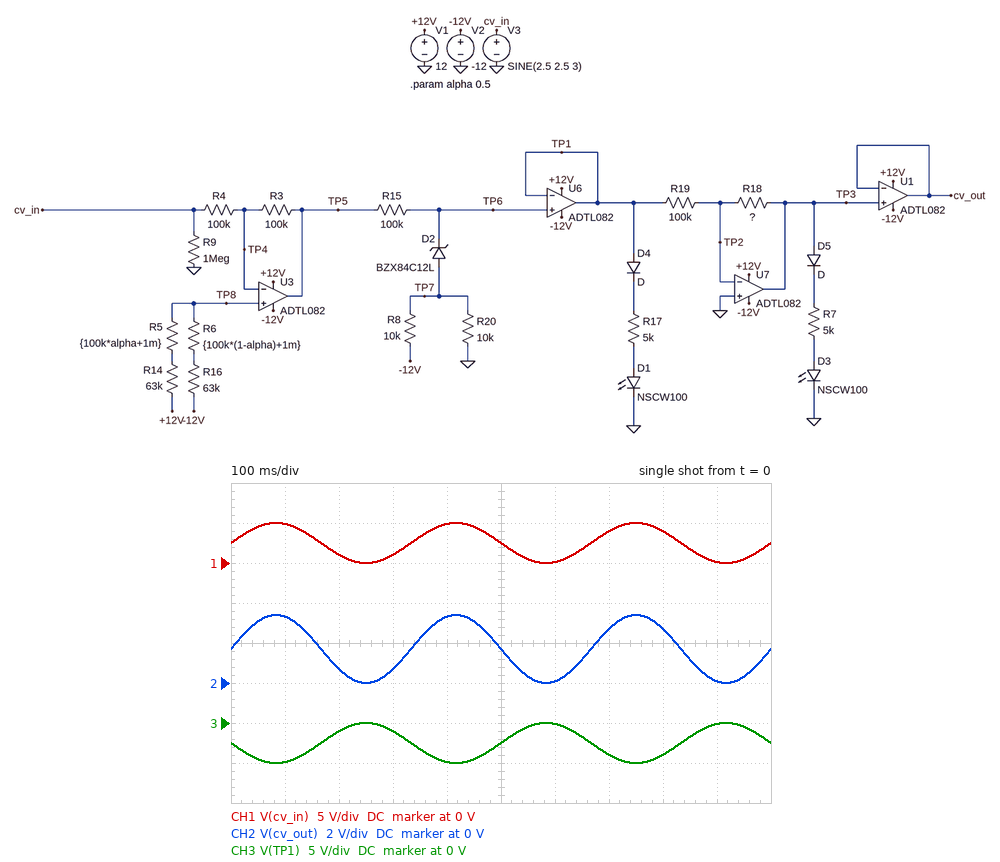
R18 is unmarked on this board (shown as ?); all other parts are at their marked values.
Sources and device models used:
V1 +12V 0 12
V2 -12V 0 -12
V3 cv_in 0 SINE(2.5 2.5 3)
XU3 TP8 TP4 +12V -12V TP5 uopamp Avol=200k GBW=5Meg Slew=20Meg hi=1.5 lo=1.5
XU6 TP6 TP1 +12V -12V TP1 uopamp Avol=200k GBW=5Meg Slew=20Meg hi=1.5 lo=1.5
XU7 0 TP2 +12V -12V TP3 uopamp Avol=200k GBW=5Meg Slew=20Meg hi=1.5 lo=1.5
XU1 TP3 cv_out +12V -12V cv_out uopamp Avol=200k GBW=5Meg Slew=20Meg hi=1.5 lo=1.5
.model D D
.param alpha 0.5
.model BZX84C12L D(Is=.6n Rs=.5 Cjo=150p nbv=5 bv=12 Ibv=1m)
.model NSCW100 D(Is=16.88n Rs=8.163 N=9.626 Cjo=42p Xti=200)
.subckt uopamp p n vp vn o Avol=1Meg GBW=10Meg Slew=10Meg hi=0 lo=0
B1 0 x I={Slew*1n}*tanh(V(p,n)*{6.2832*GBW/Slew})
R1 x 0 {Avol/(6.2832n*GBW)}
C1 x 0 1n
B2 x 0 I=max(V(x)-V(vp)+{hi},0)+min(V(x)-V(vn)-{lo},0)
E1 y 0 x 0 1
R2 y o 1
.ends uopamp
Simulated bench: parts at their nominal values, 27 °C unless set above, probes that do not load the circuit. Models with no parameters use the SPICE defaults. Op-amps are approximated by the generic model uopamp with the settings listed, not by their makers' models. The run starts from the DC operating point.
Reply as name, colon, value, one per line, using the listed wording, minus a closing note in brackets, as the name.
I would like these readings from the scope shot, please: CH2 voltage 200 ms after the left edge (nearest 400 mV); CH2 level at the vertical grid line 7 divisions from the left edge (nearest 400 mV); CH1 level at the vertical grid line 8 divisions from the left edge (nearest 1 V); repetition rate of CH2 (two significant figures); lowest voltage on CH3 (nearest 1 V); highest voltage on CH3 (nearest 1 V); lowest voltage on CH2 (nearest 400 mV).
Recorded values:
CH2 voltage 200 ms after the left edge: 800 mV
CH2 level at the vertical grid line 7 divisions from the left edge: 2.8 V
CH1 level at the vertical grid line 8 divisions from the left edge: 4 V
repetition rate of CH2: 3.0 Hz
lowest voltage on CH3: -5 V
highest voltage on CH3: 0 V
lowest voltage on CH2: 0 V
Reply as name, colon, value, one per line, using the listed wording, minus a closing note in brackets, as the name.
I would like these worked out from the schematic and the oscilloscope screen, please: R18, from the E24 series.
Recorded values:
R18, from the E24 series: 68 kΩ
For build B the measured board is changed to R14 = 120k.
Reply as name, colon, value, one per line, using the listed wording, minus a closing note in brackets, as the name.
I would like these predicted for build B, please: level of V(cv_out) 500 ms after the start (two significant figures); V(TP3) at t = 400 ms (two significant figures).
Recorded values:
level of V(cv_out) 500 ms after the start: 4.3 V
V(TP3) at t = 400 ms: 4.4 V
